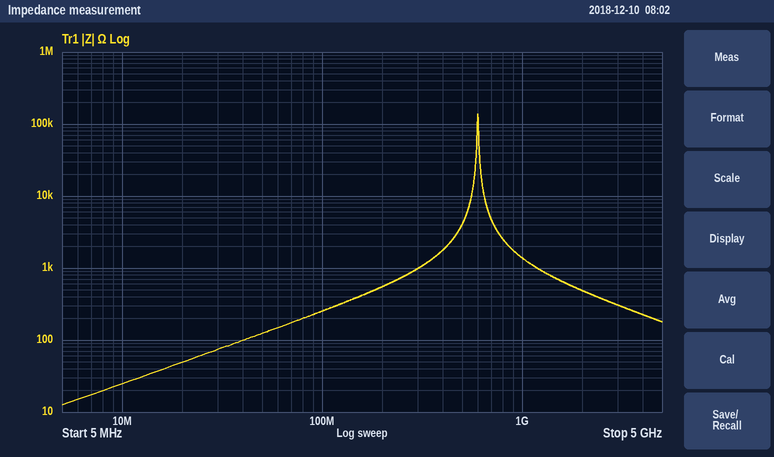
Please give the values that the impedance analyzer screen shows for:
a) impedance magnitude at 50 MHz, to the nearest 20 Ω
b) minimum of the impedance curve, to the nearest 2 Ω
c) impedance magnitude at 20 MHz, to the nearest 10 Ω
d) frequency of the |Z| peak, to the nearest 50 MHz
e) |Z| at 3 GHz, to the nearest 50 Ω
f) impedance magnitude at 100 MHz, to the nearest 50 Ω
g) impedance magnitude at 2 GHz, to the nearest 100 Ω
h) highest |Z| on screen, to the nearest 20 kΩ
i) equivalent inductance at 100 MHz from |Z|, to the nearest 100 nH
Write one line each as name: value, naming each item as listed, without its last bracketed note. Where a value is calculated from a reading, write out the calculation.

impedance magnitude at 50 MHz, to the nearest 20 Ω: 120 Ω
minimum of the impedance curve, to the nearest 2 Ω: 12 Ω
impedance magnitude at 20 MHz, to the nearest 10 Ω: 50 Ω
frequency of the |Z| peak, to the nearest 50 MHz: 600 MHz
|Z| at 3 GHz, to the nearest 50 Ω: 300 Ω
impedance magnitude at 100 MHz, to the nearest 50 Ω: 250 Ω
impedance magnitude at 2 GHz, to the nearest 100 Ω: 500 Ω
highest |Z| on screen, to the nearest 20 kΩ: 140 kΩ
equivalent inductance at 100 MHz from |Z|, to the nearest 100 nH: L = 250 Ω/(2π × 100 MHz) ≈ 398 nH, so 400 nH to the nearest 100 nH
